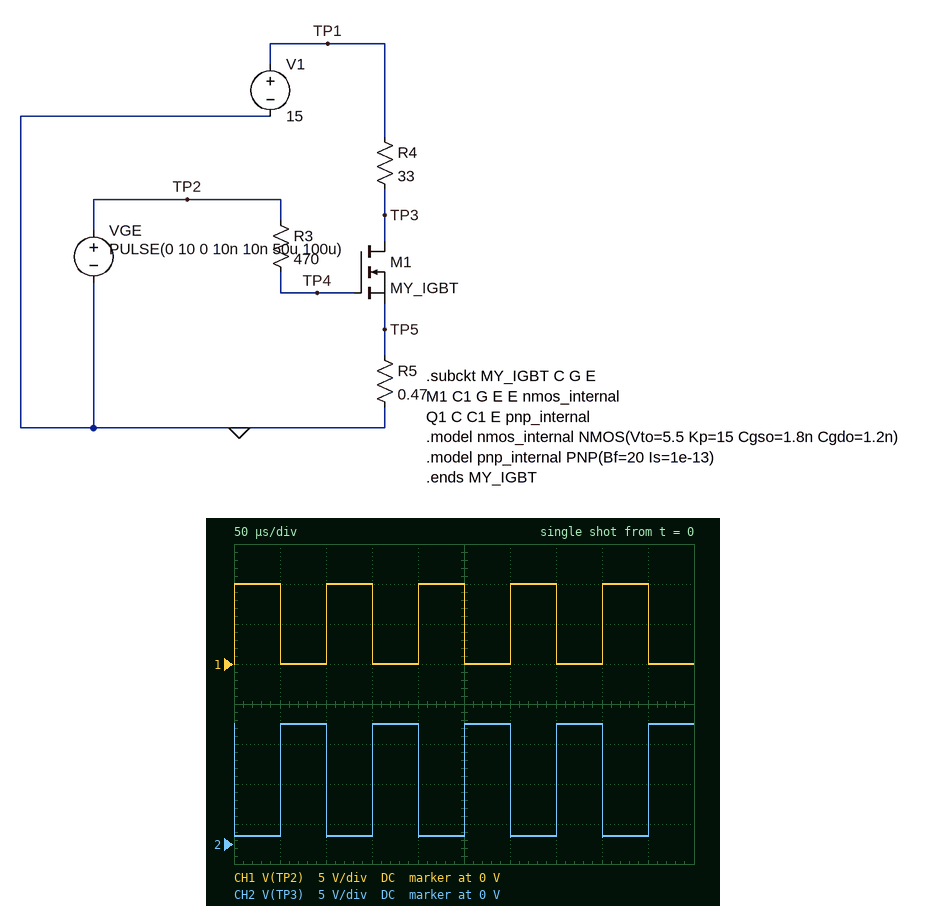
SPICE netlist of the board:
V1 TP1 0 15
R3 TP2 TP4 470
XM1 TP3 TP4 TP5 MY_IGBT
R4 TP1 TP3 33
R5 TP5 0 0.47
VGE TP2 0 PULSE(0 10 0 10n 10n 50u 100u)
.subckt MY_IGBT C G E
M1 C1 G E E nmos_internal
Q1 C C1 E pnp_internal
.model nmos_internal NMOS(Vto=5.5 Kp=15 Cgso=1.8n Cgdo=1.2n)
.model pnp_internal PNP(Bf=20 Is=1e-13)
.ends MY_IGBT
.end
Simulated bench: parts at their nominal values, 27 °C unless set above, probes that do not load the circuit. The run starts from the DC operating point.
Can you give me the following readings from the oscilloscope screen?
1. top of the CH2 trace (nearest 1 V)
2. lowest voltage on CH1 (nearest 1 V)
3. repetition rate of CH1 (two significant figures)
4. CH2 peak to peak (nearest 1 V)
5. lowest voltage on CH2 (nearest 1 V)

15 V
0 V
10 kHz
14 V
1 V
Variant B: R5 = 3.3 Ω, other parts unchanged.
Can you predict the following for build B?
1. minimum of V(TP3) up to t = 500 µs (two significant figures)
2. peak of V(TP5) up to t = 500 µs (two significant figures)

2.0 V
1.3 V
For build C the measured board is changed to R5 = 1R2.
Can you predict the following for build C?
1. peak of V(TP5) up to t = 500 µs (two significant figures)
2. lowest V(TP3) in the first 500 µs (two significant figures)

500 mV
1.2 V
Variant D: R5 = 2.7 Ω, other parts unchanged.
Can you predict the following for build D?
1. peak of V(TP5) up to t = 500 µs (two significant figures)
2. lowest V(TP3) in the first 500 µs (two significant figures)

1.1 V
1.8 V
